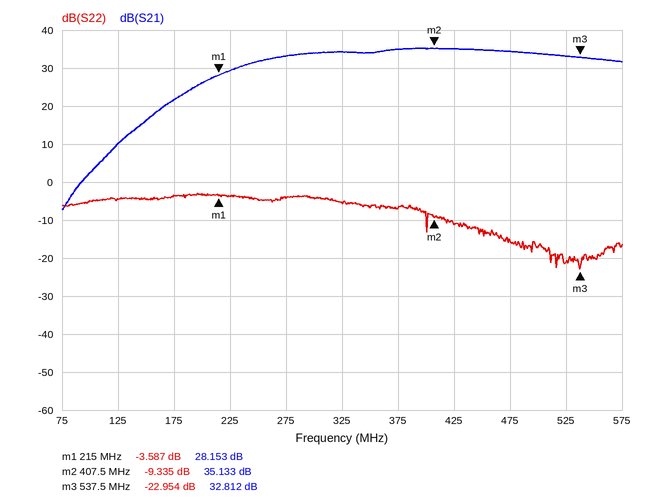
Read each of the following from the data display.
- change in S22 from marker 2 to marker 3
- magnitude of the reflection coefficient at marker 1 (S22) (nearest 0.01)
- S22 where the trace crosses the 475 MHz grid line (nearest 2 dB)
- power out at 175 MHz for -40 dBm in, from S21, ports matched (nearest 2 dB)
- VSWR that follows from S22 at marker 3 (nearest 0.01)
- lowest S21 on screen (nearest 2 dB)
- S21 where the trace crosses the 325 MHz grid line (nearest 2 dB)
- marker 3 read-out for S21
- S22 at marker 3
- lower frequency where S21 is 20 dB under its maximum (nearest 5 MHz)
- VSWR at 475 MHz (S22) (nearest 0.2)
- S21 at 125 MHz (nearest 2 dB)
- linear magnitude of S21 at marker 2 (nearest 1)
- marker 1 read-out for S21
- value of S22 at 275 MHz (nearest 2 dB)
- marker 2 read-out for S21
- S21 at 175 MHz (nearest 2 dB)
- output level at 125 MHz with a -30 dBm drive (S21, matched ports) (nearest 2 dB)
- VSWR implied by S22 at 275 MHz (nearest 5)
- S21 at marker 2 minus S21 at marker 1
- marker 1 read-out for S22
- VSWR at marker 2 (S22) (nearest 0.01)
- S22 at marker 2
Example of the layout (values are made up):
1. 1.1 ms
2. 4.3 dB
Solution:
1. -13.619 dB
2. 0.66
3. -16 dB
4. -18 dBm
5. 1.15
6. -8 dB
7. 34 dB
8. 32.812 dB
9. -22.954 dB
10. 145 MHz
11. 1.4
12. 10 dB
13. 57
14. 28.153 dB
15. -4 dB
16. 35.133 dB
17. 22 dB
18. -20 dBm
19. 5
20. 6.980 dB
21. -3.587 dB
22. 2.04
23. -9.335 dB
